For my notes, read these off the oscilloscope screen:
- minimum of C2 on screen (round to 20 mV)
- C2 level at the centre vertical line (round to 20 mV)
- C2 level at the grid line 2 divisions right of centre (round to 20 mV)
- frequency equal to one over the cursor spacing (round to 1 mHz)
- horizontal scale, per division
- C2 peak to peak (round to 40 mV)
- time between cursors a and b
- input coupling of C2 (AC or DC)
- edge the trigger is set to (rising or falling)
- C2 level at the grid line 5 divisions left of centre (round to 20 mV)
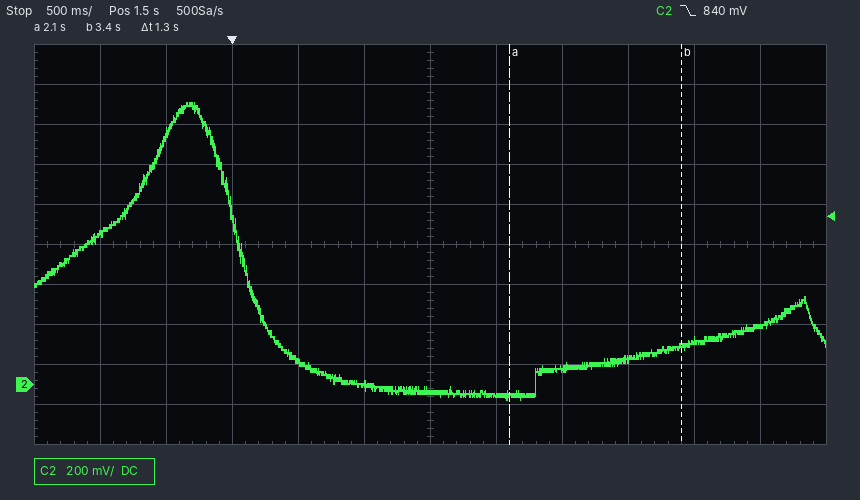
-80 mV
-40 mV
80 mV
769 mHz
500 ms
1.48 V
1.3 s
DC
falling
760 mV
